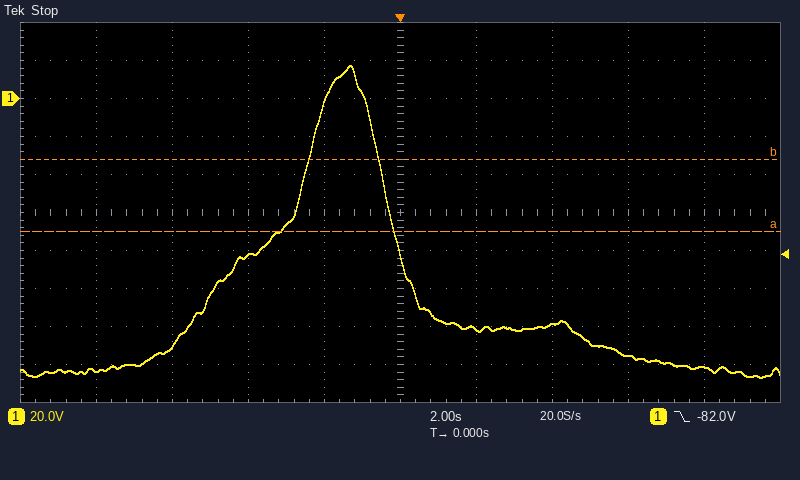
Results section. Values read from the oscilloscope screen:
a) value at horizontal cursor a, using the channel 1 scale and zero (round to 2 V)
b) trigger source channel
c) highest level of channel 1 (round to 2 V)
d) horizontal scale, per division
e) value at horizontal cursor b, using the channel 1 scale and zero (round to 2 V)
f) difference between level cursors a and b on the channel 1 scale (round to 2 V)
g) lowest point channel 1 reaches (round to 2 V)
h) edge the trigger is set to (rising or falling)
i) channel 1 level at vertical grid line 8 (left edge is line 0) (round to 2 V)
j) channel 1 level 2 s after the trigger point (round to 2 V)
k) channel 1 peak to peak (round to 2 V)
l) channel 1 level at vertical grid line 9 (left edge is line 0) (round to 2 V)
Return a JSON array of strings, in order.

["-70 V", "channel 1", "18 V", "2 s", "-32 V", "38 V", "-146 V", "falling", "-136 V", "-122 V", "164 V", "-142 V"]
